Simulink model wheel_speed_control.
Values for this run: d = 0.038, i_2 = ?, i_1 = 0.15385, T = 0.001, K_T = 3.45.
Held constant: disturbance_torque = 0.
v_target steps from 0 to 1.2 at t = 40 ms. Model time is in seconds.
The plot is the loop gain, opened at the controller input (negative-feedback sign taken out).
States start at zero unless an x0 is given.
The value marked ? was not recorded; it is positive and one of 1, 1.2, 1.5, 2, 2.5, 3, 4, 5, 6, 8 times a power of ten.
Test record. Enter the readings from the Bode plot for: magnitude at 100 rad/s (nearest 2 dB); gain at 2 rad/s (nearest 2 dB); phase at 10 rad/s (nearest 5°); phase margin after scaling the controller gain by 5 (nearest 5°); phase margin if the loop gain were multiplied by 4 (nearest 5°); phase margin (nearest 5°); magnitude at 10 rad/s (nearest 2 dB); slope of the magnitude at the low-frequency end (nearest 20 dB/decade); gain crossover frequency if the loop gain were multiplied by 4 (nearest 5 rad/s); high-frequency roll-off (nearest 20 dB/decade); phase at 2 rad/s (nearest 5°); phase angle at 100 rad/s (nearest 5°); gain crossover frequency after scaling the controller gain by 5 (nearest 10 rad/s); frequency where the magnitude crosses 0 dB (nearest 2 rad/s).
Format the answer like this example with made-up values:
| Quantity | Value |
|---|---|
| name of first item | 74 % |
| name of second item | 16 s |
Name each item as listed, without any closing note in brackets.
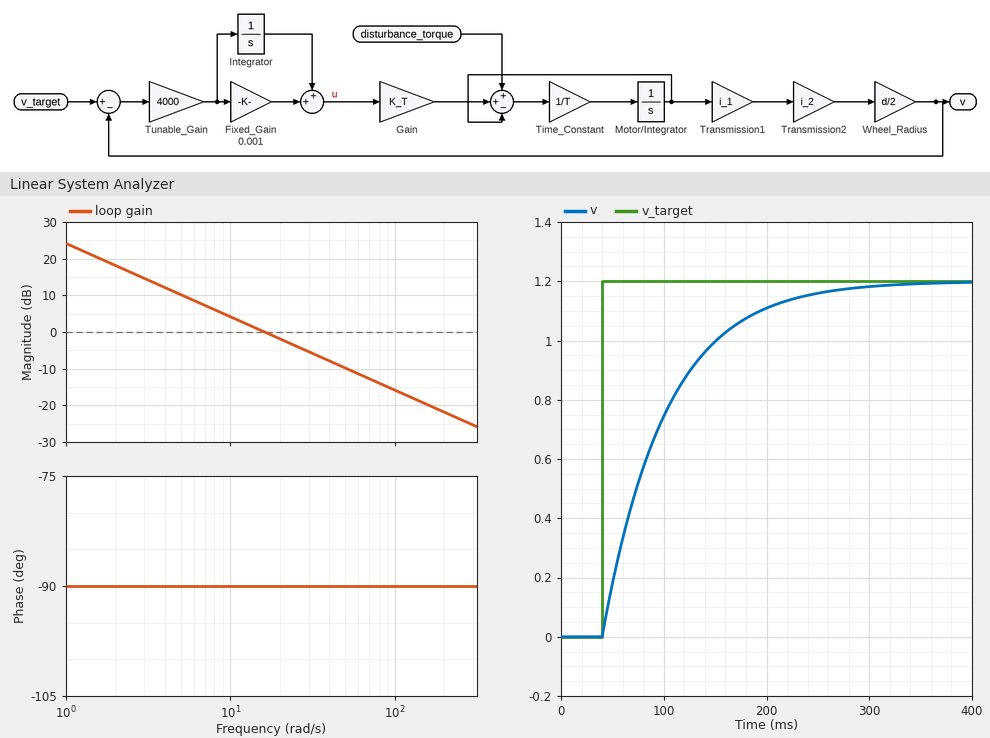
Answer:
| Quantity | Value |
|---|---|
| magnitude at 100 rad/s | -16 dB |
| gain at 2 rad/s | 18 dB |
| phase at 10 rad/s | -90° |
| phase margin after scaling the controller gain by 5 | 90° |
| phase margin if the loop gain were multiplied by 4 | 90° |
| phase margin | 90° |
| magnitude at 10 rad/s | 4 dB |
| slope of the magnitude at the low-frequency end | -20 dB/decade |
| gain crossover frequency if the loop gain were multiplied by 4 | 65 rad/s |
| high-frequency roll-off | -20 dB/decade |
| phase at 2 rad/s | -90° |
| phase angle at 100 rad/s | -90° |
| gain crossover frequency after scaling the controller gain by 5 | 80 rad/s |
| frequency where the magnitude crosses 0 dB | 16 rad/s |
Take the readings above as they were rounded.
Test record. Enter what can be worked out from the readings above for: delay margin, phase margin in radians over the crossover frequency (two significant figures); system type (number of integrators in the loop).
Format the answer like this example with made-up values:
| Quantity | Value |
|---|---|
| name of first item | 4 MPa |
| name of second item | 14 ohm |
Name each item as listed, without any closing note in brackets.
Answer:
| Quantity | Value |
|---|---|
| delay margin, phase margin in radians over the crossover frequency | 0.098 s |
| system type | 1 |
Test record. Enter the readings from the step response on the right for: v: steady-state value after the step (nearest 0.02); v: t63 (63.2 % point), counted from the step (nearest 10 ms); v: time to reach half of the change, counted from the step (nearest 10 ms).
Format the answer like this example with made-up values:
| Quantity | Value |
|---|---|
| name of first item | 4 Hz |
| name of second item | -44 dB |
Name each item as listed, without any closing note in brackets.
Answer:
| Quantity | Value |
|---|---|
| v: steady-state value after the step | 1.20 |
| v: t63 (63.2 % point), counted from the step | 60 ms |
| v: time to reach half of the change, counted from the step | 40 ms |
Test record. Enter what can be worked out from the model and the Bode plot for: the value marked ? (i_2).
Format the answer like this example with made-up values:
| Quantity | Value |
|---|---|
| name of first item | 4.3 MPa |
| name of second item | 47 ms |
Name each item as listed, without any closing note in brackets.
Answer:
| Quantity | Value |
|---|---|
| the value marked ? | 0.4 |
